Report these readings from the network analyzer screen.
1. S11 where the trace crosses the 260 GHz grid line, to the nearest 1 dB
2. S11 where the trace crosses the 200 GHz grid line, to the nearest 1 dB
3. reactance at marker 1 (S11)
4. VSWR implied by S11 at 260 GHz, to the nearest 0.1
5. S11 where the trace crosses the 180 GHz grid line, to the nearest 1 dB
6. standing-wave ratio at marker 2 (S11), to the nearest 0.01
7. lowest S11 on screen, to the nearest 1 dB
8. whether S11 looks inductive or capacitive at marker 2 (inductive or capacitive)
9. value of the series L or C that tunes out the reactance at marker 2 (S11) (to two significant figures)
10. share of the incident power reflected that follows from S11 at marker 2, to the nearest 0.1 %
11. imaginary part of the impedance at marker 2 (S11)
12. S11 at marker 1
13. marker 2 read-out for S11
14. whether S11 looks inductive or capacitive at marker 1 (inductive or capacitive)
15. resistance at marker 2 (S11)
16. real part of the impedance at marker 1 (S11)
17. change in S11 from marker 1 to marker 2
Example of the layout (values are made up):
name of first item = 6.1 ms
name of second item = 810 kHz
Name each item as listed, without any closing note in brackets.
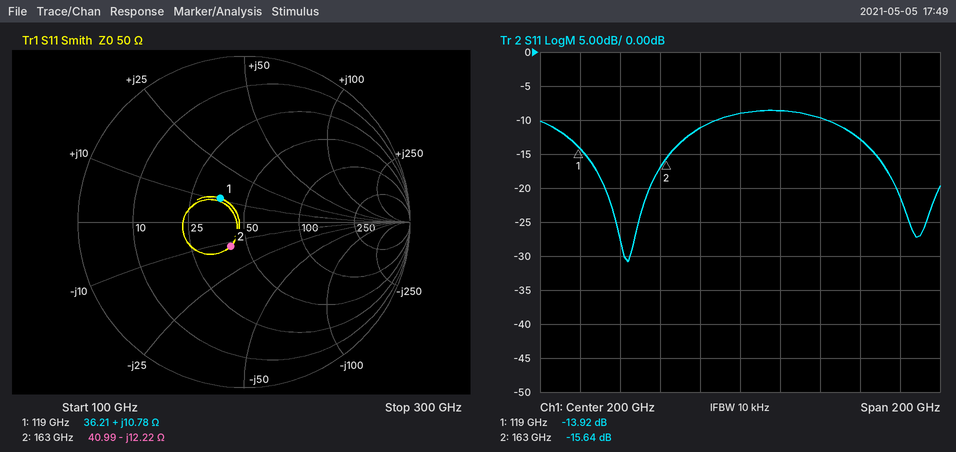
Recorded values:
S11 where the trace crosses the 260 GHz grid line, to the nearest 1 dB = -13 dB
S11 where the trace crosses the 200 GHz grid line, to the nearest 1 dB = -9 dB
reactance at marker 1 = +10.78 Ω
VSWR implied by S11 at 260 GHz, to the nearest 0.1 = 1.6
S11 where the trace crosses the 180 GHz grid line, to the nearest 1 dB = -11 dB
standing-wave ratio at marker 2 (S11), to the nearest 0.01 = 1.40
lowest S11 on screen, to the nearest 1 dB = -31 dB
whether S11 looks inductive or capacitive at marker 2 = capacitive
value of the series L or C that tunes out the reactance at marker 2 (S11) = 12 pH
share of the incident power reflected that follows from S11 at marker 2, to the nearest 0.1 % = 2.7 %
imaginary part of the impedance at marker 2 = -12.22 Ω
S11 at marker 1 = -13.92 dB
marker 2 read-out for S11 = -15.64 dB
whether S11 looks inductive or capacitive at marker 1 = inductive
resistance at marker 2 = 40.99 Ω
real part of the impedance at marker 1 = 36.21 Ω
change in S11 from marker 1 to marker 2 = -1.72 dB
